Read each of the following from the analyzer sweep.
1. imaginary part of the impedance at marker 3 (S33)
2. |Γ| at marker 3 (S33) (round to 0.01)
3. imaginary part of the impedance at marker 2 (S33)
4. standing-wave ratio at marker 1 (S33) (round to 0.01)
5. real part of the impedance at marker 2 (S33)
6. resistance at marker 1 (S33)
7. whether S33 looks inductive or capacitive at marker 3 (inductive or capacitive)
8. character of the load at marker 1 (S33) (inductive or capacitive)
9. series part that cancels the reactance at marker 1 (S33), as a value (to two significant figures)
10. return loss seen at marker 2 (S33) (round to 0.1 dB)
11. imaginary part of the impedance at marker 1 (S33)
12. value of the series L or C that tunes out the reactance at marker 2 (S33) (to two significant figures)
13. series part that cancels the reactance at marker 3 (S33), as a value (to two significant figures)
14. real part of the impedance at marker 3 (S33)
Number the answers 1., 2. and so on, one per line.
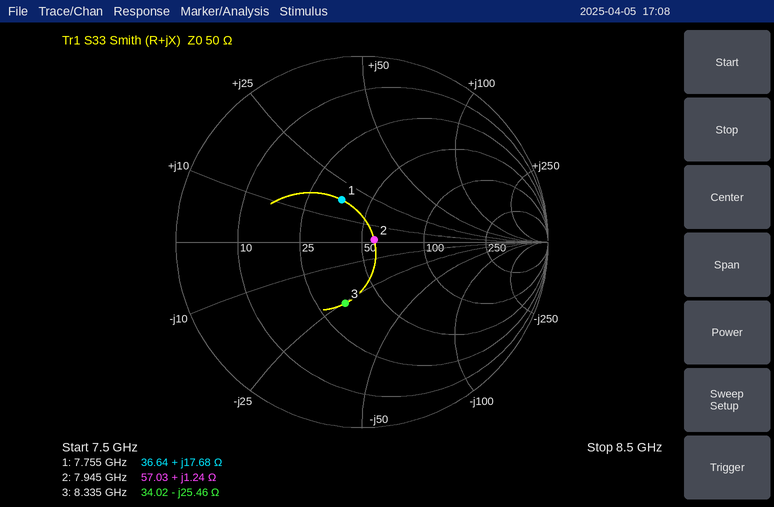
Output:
1. -25.46 Ω
2. 0.34
3. +1.24 Ω
4. 1.67
5. 57.03 Ω
6. 36.64 Ω
7. capacitive
8. inductive
9. 1.2 pF
10. 23.5 dB
11. +17.68 Ω
12. 16 pF
13. 490 pH
14. 34.02 Ω
